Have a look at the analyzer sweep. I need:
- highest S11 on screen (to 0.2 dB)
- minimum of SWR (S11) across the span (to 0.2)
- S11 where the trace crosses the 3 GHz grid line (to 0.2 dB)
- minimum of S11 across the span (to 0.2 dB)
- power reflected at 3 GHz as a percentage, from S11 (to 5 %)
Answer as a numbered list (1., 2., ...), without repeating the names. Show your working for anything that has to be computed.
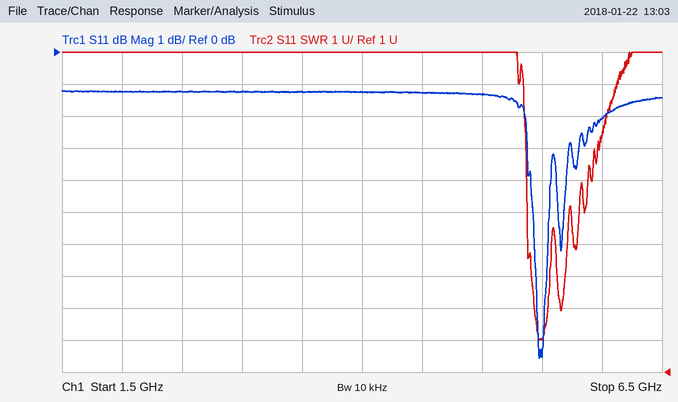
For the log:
1. -1.2 dB
2. 2.0
3. -1.2 dB
4. -9.6 dB
5. 10^(-1.2/10) ≈ 75.9 %, so 75 % to the nearest 5 %
